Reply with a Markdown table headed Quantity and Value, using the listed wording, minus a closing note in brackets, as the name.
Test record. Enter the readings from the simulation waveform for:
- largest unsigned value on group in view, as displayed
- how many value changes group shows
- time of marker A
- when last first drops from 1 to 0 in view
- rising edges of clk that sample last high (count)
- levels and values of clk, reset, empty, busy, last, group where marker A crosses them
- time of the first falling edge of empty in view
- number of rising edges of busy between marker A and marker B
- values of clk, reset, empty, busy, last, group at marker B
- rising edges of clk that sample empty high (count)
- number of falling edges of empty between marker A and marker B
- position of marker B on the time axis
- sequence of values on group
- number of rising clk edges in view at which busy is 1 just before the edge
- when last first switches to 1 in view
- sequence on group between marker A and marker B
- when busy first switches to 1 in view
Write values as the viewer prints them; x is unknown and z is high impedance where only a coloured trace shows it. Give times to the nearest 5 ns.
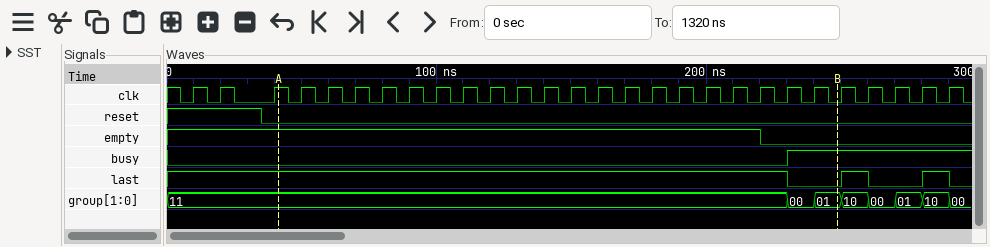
| Quantity | Value |
|---|---|
| largest unsigned value on group in view, as displayed | 11 |
| how many value changes group shows | 7 |
| time of marker A | 40 ns |
| when last first drops from 1 to 0 in view | 230 ns |
| rising edges of clk that sample last high | 24 |
| levels and values of clk, reset, empty, busy, last, group where marker A crosses them | clk=1, reset=0, empty=1, busy=0, last=1, group=11 |
| time of the first falling edge of empty in view | 220 ns |
| number of rising edges of busy between marker A and marker B | 1 |
| values of clk, reset, empty, busy, last, group at marker B | clk=0, reset=0, empty=0, busy=1, last=0, group=01 |
| rising edges of clk that sample empty high | 21 |
| number of falling edges of empty between marker A and marker B | 1 |
| position of marker B on the time axis | 250 ns |
| sequence of values on group | 11, 00, 01, 10, 00, 01, 10, 00 |
| number of rising clk edges in view at which busy is 1 just before the edge | 6 |
| when last first switches to 1 in view | 250 ns |
| sequence on group between marker A and marker B | 11, 00, 01 |
| when busy first switches to 1 in view | 230 ns |
